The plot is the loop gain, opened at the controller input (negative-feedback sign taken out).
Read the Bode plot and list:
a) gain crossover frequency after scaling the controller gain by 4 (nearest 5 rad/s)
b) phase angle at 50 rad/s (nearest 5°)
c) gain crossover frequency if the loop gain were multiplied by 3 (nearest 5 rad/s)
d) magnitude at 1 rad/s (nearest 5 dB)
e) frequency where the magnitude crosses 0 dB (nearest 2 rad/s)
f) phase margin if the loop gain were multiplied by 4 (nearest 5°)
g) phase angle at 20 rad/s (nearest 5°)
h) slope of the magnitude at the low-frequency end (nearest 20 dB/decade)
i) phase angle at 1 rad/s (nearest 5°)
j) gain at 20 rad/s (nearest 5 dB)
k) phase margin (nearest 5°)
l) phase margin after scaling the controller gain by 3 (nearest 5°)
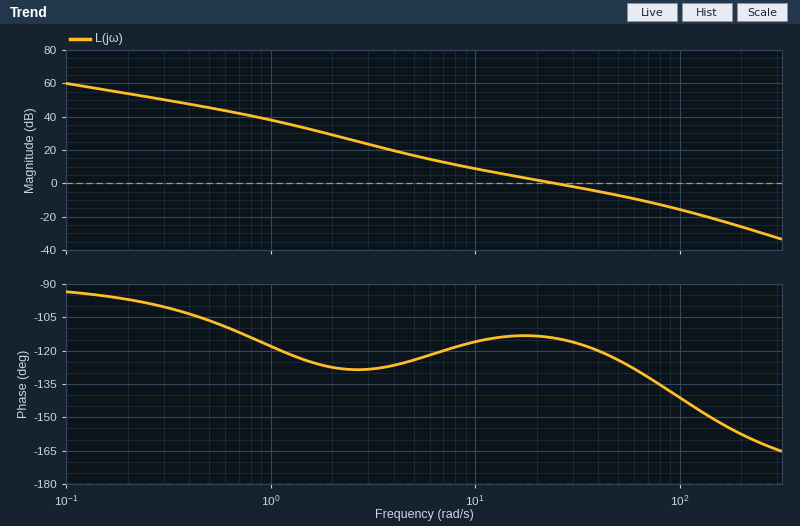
75 rad/s
-125°
60 rad/s
40 dB
24 rad/s
45°
-115°
-20 dB/decade
-120°
0 dB
65°
50°
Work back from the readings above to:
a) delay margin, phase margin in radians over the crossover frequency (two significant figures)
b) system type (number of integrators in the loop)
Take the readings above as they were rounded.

0.047 s
1
